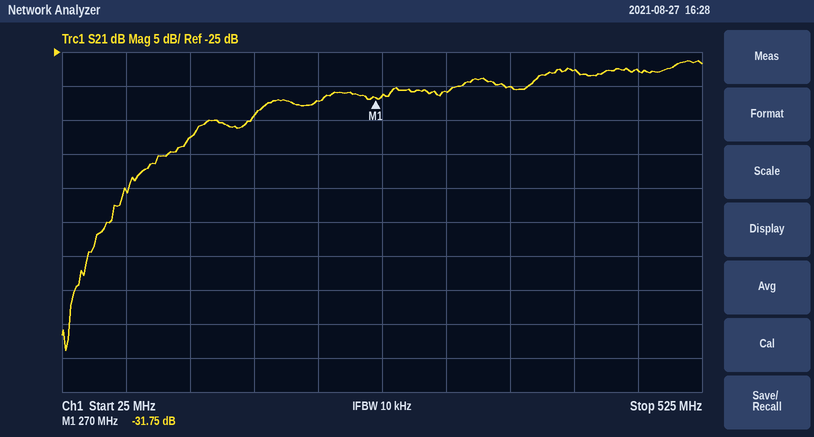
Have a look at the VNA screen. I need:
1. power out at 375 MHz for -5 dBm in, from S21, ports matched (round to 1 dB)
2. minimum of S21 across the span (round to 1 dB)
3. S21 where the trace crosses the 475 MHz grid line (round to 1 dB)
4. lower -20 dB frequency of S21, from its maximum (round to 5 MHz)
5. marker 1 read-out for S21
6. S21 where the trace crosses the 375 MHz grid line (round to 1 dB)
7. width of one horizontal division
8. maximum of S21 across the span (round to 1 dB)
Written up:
-35 dBm
-69 dB
-28 dB
70 MHz
-31.75 dB
-30 dB
50 MHz
-26 dB
